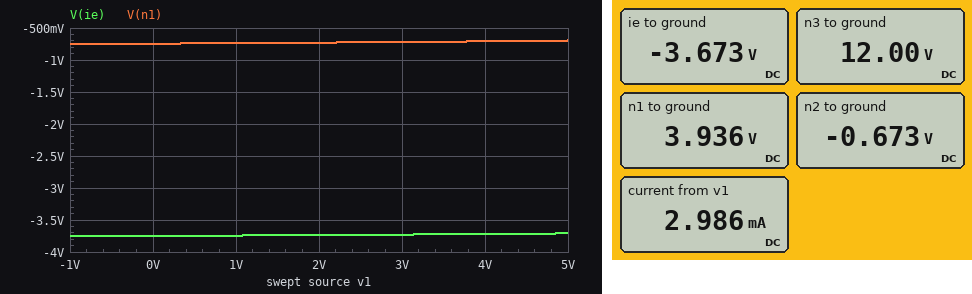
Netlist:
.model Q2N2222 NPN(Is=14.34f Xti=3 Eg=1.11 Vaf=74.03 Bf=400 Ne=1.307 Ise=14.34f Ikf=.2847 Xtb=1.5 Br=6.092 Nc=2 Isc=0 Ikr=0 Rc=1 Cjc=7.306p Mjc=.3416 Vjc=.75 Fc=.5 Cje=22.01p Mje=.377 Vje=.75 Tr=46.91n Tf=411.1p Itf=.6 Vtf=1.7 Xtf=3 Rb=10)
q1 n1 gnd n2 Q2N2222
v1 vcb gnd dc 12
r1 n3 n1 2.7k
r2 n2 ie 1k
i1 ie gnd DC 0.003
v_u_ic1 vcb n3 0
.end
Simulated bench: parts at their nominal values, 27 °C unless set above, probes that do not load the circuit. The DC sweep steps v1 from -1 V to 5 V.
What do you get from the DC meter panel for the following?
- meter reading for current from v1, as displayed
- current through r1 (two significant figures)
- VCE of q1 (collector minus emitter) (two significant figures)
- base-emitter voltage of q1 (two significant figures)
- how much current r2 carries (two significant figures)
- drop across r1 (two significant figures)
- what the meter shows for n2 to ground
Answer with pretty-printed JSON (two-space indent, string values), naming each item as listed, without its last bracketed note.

{
  "meter reading for current from v1, as displayed": "2.986 mA",
  "current through r1": "3.0 mA",
  "VCE of q1 (collector minus emitter)": "4.6 V",
  "base-emitter voltage of q1": "670 mV",
  "how much current r2 carries": "3.0 mA",
  "drop across r1": "8.1 V",
  "what the meter shows for n2 to ground": "-0.673 V"
}
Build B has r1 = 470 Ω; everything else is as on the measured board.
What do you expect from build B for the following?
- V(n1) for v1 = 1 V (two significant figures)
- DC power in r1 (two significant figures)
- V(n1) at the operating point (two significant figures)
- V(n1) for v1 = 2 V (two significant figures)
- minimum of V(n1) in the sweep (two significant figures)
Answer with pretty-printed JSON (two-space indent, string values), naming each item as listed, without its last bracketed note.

{
  "V(n1) for v1 = 1 V": "-400 mV",
  "DC power in r1": "4.2 mW",
  "V(n1) at the operating point": "11 V",
  "V(n1) for v1 = 2 V": "600 mV",
  "minimum of V(n1) in the sweep": "-760 mV"
}
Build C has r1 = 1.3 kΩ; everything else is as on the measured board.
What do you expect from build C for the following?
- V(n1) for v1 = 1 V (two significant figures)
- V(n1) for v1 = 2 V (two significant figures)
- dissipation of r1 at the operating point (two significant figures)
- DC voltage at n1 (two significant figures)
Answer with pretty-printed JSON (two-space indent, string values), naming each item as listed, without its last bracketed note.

{
  "V(n1) for v1 = 1 V": "-720 mV",
  "V(n1) for v1 = 2 V": "-700 mV",
  "dissipation of r1 at the operating point": "12 mW",
  "DC voltage at n1": "8.1 V"
}
